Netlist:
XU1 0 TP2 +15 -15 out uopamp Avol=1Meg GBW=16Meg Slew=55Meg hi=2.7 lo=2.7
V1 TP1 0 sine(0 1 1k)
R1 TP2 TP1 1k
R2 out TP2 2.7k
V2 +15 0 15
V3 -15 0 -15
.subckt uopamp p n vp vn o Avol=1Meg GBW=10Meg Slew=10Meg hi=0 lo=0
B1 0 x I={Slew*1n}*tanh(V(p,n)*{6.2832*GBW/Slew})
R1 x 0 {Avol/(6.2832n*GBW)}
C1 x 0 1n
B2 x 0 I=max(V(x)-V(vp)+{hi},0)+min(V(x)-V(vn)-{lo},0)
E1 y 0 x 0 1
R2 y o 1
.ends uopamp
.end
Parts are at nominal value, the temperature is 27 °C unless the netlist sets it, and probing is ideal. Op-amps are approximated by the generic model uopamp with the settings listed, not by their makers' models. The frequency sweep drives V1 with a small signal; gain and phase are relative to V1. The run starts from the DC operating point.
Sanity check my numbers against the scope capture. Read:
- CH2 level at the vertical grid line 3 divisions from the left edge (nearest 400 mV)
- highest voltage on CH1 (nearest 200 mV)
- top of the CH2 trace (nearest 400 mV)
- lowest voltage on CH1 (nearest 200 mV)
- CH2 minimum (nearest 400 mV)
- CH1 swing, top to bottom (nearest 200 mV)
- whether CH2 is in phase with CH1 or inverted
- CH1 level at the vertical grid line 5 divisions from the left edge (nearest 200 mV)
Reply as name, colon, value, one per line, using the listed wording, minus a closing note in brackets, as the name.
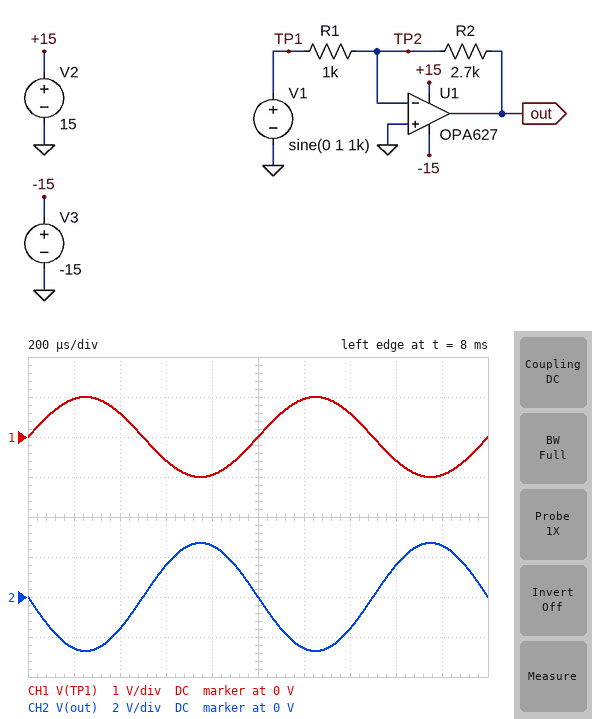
CH2 level at the vertical grid line 3 divisions from the left edge: 1.6 V
highest voltage on CH1: 1.0 V
top of the CH2 trace: 2.8 V
lowest voltage on CH1: -1.0 V
CH2 minimum: -2.8 V
CH1 swing, top to bottom: 2.0 V
whether CH2 is in phase with CH1 or inverted: inverted
CH1 level at the vertical grid line 5 divisions from the left edge: 0 V
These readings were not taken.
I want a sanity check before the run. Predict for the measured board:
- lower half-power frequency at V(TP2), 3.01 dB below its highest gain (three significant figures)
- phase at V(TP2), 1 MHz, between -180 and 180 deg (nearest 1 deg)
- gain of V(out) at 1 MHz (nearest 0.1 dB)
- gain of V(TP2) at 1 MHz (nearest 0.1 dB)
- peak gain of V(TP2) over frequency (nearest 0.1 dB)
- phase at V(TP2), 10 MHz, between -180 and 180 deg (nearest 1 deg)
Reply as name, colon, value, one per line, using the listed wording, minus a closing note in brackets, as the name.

lower half-power frequency at V(TP2), 3.01 dB below its highest gain: 4.32 MHz
phase at V(TP2), 1 MHz, between -180 and 180 deg: 77 deg
gain of V(out) at 1 MHz: 8.4 dB
gain of V(TP2) at 1 MHz: -15.7 dB
peak gain of V(TP2) over frequency: -2.7 dB
phase at V(TP2), 10 MHz, between -180 and 180 deg: 23 deg
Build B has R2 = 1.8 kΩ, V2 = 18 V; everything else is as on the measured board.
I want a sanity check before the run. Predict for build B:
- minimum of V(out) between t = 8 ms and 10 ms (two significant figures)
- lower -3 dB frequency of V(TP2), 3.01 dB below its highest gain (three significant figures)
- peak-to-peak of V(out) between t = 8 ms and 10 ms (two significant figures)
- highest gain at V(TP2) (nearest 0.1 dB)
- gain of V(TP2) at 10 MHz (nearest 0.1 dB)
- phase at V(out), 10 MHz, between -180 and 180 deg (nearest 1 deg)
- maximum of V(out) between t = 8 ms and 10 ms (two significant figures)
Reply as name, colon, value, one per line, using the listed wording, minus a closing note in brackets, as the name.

minimum of V(out) between t = 8 ms and 10 ms: -1.8 V
lower -3 dB frequency of V(TP2), 3.01 dB below its highest gain: 5.71 MHz
peak-to-peak of V(out) between t = 8 ms and 10 ms: 3.6 V
highest gain at V(TP2): -3.8 dB
gain of V(TP2) at 10 MHz: -5.1 dB
phase at V(out), 10 MHz, between -180 and 180 deg: 120 deg
maximum of V(out) between t = 8 ms and 10 ms: 1.8 V
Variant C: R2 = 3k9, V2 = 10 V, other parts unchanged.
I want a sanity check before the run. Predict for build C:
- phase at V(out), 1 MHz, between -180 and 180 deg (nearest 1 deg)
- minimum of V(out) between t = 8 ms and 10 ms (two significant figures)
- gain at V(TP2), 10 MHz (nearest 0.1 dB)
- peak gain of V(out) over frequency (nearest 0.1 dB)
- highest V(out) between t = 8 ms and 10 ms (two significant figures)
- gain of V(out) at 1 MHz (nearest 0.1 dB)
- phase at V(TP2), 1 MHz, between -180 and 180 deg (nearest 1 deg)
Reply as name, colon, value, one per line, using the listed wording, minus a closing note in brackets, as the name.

phase at V(out), 1 MHz, between -180 and 180 deg: 163 deg
minimum of V(out) between t = 8 ms and 10 ms: -3.9 V
gain at V(TP2), 10 MHz: -2.4 dB
peak gain of V(out) over frequency: 11.8 dB
highest V(out) between t = 8 ms and 10 ms: 3.9 V
gain of V(out) at 1 MHz: 11.4 dB
phase at V(TP2), 1 MHz, between -180 and 180 deg: 73 deg
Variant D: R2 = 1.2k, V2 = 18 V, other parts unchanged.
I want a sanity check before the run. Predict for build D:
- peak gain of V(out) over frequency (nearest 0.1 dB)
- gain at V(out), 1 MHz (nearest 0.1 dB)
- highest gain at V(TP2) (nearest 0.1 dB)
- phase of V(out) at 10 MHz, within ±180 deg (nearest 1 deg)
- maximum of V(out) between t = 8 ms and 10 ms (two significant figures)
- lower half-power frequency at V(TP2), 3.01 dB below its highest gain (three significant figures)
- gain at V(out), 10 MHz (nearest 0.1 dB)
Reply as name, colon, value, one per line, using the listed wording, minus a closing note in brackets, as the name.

peak gain of V(out) over frequency: 1.6 dB
gain at V(out), 1 MHz: 1.5 dB
highest gain at V(TP2): -5.3 dB
phase of V(out) at 10 MHz, within ±180 deg: 126 deg
maximum of V(out) between t = 8 ms and 10 ms: 1.2 V
lower half-power frequency at V(TP2), 3.01 dB below its highest gain: 7.27 MHz
gain at V(out), 10 MHz: -3.0 dB
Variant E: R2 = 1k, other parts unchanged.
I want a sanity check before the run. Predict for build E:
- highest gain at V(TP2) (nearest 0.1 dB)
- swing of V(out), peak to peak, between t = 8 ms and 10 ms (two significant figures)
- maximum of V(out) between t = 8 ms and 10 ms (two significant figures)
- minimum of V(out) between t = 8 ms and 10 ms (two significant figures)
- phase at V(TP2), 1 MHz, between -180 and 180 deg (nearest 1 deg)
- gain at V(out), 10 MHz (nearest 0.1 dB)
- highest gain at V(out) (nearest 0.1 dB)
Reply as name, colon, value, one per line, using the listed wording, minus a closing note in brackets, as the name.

highest gain at V(TP2): -6.0 dB
swing of V(out), peak to peak, between t = 8 ms and 10 ms: 2.0 V
maximum of V(out) between t = 8 ms and 10 ms: 1.0 V
minimum of V(out) between t = 8 ms and 10 ms: -1.0 V
phase at V(TP2), 1 MHz, between -180 and 180 deg: 83 deg
gain at V(out), 10 MHz: -4.1 dB
highest gain at V(out): 0 dB
